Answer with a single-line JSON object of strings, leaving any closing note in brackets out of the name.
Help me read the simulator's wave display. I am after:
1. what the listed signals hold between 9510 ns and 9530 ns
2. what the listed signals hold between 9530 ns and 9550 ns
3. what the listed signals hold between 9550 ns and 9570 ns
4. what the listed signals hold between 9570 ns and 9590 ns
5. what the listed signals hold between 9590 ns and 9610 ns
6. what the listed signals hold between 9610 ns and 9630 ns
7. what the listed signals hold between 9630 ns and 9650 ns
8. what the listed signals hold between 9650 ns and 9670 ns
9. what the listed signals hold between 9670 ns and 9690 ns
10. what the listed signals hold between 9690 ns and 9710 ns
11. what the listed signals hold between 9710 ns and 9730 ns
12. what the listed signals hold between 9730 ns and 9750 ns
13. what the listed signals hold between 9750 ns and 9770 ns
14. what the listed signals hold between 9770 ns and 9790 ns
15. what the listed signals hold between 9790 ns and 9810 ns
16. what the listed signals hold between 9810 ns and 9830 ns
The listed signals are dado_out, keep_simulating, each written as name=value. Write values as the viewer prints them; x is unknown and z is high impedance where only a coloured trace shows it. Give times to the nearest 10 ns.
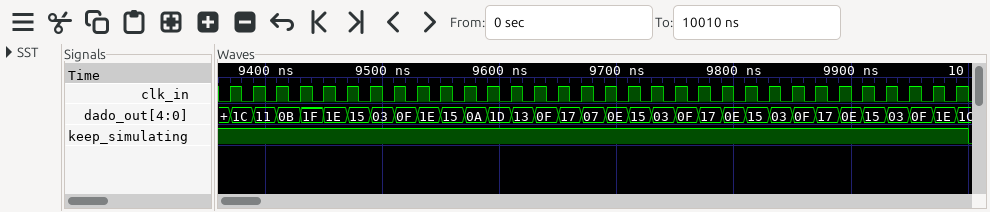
{"what the listed signals hold between 9510 ns and 9530 ns": "dado_out=0F, keep_simulating=1", "what the listed signals hold between 9530 ns and 9550 ns": "dado_out=1E, keep_simulating=1", "what the listed signals hold between 9550 ns and 9570 ns": "dado_out=15, keep_simulating=1", "what the listed signals hold between 9570 ns and 9590 ns": "dado_out=0A, keep_simulating=1", "what the listed signals hold between 9590 ns and 9610 ns": "dado_out=1D, keep_simulating=1", "what the listed signals hold between 9610 ns and 9630 ns": "dado_out=13, keep_simulating=1", "what the listed signals hold between 9630 ns and 9650 ns": "dado_out=0F, keep_simulating=1", "what the listed signals hold between 9650 ns and 9670 ns": "dado_out=17, keep_simulating=1", "what the listed signals hold between 9670 ns and 9690 ns": "dado_out=07, keep_simulating=1", "what the listed signals hold between 9690 ns and 9710 ns": "dado_out=0E, keep_simulating=1", "what the listed signals hold between 9710 ns and 9730 ns": "dado_out=15, keep_simulating=1", "what the listed signals hold between 9730 ns and 9750 ns": "dado_out=03, keep_simulating=1", "what the listed signals hold between 9750 ns and 9770 ns": "dado_out=0F, keep_simulating=1", "what the listed signals hold between 9770 ns and 9790 ns": "dado_out=17, keep_simulating=1", "what the listed signals hold between 9790 ns and 9810 ns": "dado_out=0E, keep_simulating=1", "what the listed signals hold between 9810 ns and 9830 ns": "dado_out=15, keep_simulating=1"}
